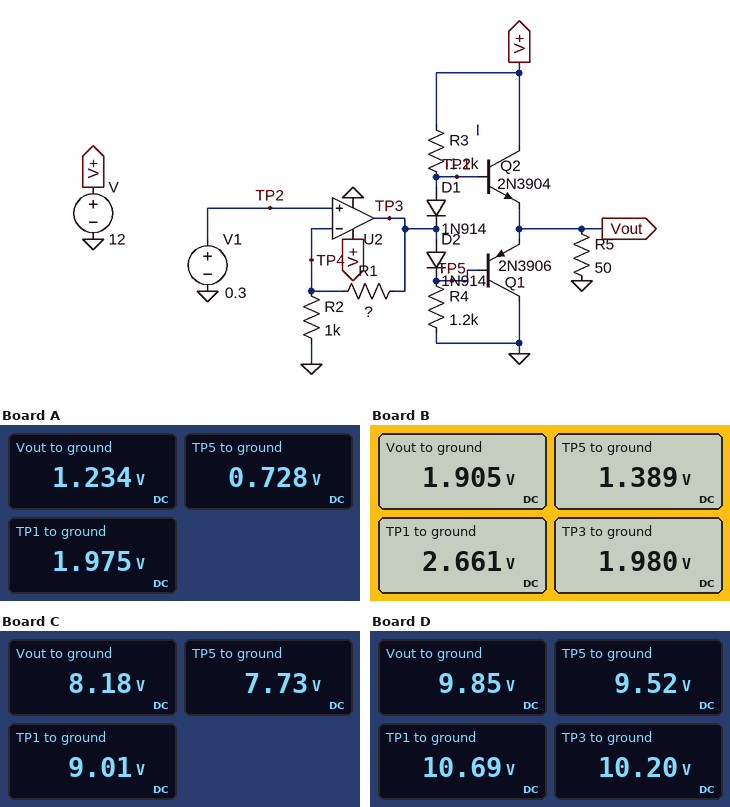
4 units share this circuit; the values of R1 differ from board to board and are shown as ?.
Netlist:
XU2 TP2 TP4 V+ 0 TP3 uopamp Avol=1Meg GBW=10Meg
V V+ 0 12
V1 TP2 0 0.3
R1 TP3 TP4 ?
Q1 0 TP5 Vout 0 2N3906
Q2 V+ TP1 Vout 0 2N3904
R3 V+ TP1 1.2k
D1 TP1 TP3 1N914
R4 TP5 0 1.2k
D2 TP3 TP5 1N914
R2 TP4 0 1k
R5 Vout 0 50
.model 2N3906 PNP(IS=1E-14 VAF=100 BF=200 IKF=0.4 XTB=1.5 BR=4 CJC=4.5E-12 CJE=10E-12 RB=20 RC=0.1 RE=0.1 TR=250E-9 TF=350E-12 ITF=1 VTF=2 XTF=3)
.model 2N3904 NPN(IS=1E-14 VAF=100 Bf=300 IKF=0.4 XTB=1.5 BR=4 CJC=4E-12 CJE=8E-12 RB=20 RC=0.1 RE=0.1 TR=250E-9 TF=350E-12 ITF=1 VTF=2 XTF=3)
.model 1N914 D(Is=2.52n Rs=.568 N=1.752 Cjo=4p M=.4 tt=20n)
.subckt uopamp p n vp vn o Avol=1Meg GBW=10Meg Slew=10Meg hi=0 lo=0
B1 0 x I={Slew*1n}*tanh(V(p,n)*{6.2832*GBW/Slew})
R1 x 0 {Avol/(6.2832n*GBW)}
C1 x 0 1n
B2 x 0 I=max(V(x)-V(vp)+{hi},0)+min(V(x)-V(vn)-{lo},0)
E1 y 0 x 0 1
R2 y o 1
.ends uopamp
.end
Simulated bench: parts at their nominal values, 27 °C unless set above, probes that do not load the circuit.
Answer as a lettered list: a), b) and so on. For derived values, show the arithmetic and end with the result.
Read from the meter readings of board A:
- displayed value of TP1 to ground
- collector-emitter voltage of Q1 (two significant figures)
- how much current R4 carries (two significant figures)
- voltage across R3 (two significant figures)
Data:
a) 1.975 V
b) 0 V - 1.234 V = -1.2 V
c) (728 mV) / 1.2 kΩ = 610 µA
d) 12 V - 1.975 V = 10 V
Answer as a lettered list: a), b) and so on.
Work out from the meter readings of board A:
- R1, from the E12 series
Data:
a) 3.3 kΩ
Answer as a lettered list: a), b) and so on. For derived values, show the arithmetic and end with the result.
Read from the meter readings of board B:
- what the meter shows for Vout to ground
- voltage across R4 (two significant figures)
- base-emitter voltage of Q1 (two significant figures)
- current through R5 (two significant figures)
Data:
a) 1.905 V
b) 1.389 V = 1.4 V
c) 1.389 V - 1.905 V = -520 mV
d) (1.905 V) / 50 Ω = 38 mA
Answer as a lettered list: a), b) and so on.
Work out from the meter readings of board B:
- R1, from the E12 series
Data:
a) 5.6 kΩ
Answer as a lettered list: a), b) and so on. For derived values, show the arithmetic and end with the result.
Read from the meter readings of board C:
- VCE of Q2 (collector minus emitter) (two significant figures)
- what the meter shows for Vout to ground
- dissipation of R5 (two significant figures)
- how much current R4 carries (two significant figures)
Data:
a) 12 V - 8.18 V = 3.8 V
b) 8.18 V
c) (8.18 V)^2 / 50 Ω = 1.3 W
d) (7.73 V) / 1.2 kΩ = 6.4 mA
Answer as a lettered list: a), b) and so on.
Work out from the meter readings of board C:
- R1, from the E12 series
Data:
a) 27 kΩ
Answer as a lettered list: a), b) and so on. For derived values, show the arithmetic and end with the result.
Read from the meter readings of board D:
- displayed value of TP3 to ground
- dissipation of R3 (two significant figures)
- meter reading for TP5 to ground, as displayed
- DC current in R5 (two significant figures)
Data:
a) 10.20 V
b) (12 V - 10.69 V)^2 / 1.2 kΩ = 1.4 mW
c) 9.52 V
d) (9.85 V) / 50 Ω = 200 mA
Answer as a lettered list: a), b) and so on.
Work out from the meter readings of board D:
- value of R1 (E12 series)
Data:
a) 33 kΩ
